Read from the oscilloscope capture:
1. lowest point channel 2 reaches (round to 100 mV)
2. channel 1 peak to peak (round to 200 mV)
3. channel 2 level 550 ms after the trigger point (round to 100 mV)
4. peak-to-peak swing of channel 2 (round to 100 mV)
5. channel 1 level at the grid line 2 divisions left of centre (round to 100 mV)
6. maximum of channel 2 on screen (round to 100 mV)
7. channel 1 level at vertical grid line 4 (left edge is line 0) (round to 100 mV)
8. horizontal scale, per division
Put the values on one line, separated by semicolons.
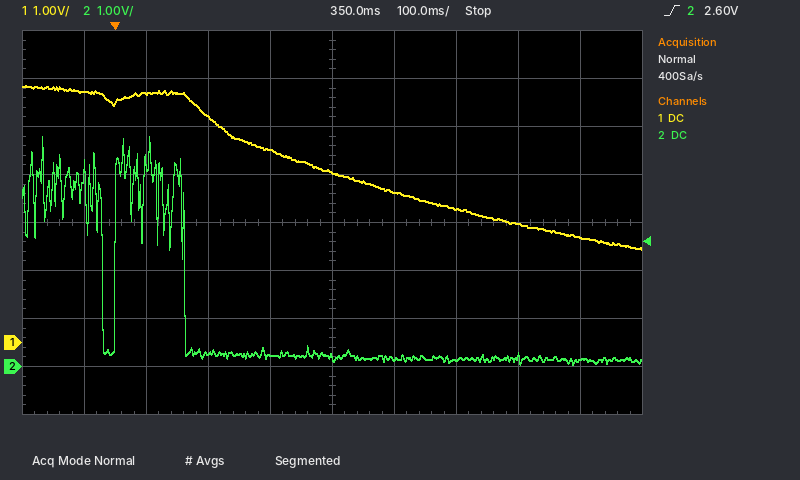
0.0 V; 3.4 V; 100 mV; 4.8 V; 4.7 V; 4.8 V; 4.0 V; 100 ms
